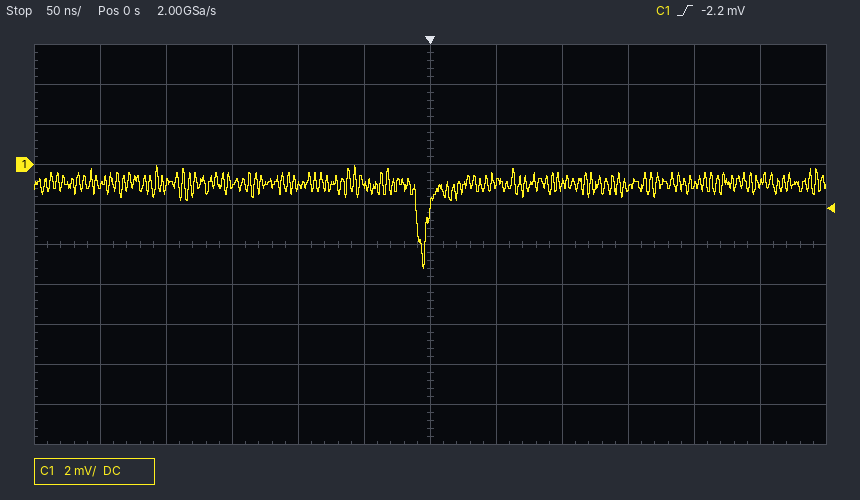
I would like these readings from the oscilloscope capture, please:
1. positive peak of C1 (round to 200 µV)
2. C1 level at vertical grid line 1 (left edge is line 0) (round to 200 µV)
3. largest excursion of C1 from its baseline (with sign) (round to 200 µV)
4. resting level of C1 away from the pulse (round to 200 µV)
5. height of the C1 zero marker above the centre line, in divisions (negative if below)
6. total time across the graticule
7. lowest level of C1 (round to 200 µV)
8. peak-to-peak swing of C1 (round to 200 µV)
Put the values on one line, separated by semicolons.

0.0 mV; -1.0 mV; -4.2 mV; -1.0 mV; +2.0 div; 600 ns; -5.2 mV; 5.2 mV
